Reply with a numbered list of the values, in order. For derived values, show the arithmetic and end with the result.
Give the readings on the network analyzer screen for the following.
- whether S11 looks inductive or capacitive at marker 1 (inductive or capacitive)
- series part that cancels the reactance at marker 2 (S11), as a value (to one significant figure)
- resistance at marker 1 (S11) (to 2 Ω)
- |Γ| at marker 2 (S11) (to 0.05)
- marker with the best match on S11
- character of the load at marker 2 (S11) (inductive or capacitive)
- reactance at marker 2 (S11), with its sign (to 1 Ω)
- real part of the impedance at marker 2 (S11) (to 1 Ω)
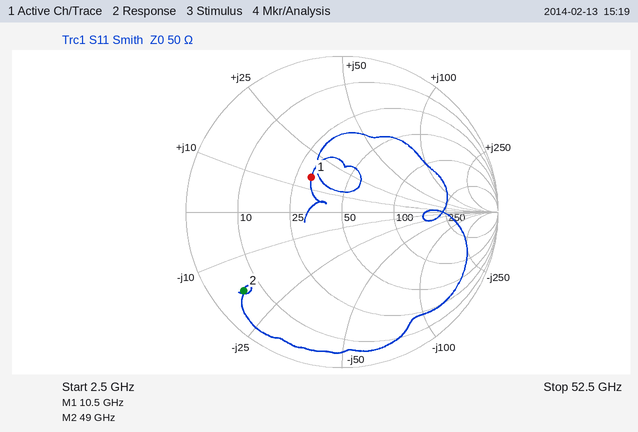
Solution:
1. inductive
2. L = 17 Ω/(2π × 49 GHz) ≈ 55.2 pH, so 60 pH to one significant figure
3. 30 Ω
4. 0.80
5. marker 1
6. capacitive
7. -17 Ω
8. 6 Ω
